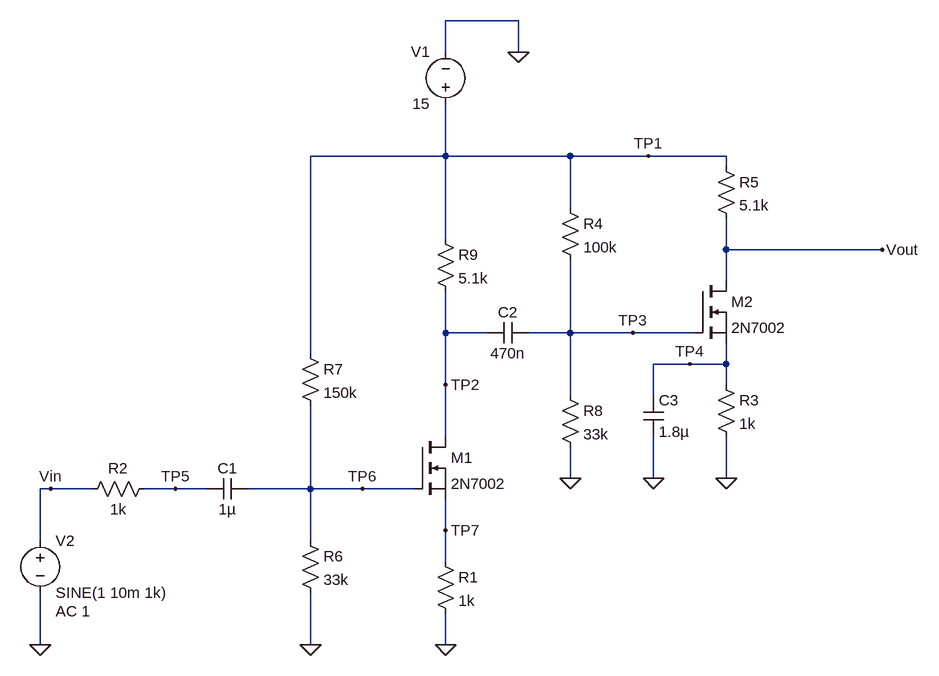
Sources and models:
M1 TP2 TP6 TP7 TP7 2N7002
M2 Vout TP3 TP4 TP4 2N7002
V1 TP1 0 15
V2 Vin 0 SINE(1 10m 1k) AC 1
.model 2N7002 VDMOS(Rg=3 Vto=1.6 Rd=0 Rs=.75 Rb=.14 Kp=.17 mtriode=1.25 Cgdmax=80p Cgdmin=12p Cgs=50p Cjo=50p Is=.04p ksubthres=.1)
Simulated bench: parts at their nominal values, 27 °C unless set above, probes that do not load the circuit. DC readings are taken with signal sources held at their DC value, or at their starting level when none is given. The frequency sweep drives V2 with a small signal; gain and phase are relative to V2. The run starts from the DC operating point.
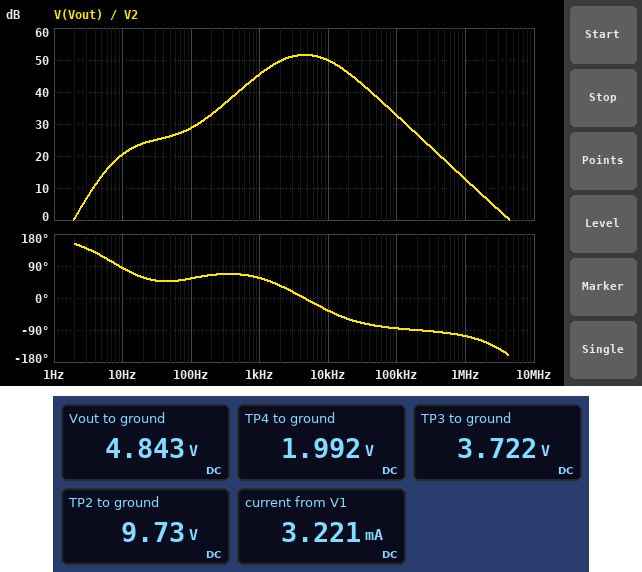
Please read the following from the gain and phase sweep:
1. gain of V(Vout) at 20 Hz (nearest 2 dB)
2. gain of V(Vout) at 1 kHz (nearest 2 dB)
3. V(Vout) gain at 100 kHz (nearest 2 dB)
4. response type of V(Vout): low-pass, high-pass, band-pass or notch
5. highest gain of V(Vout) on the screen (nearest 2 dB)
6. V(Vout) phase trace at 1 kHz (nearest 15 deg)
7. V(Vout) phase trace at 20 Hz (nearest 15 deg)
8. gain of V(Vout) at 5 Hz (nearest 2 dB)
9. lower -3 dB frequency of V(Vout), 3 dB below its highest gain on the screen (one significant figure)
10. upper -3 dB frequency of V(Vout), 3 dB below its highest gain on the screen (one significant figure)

24 dB
46 dB
32 dB
band-pass
52 dB
60 deg
60 deg
14 dB
2 kHz
10 kHz
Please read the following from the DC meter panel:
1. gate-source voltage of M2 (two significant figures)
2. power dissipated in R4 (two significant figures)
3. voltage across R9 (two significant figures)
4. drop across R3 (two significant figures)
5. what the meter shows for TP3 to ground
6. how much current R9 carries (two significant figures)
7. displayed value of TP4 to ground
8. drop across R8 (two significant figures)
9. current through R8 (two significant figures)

1.7 V
1.3 mW
5.3 V
2.0 V
3.722 V
1.0 mA
1.992 V
3.7 V
110 µA
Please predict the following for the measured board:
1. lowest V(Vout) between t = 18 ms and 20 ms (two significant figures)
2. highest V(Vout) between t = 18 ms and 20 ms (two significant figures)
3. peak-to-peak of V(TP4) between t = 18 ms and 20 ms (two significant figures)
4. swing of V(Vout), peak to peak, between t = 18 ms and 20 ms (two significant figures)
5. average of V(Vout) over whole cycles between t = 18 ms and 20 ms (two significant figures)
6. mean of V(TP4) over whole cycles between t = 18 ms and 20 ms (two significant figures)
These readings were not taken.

2.9 V
6.7 V
66 mV
3.8 V
4.8 V
2.0 V
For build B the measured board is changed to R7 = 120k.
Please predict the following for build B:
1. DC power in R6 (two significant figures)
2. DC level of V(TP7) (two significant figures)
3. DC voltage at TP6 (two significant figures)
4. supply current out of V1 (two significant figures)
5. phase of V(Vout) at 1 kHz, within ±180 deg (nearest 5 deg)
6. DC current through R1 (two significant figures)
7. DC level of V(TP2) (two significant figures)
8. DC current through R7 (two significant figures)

320 µW
1.5 V
3.2 V
3.7 mA
55 deg
1.5 mA
7.2 V
98 µA
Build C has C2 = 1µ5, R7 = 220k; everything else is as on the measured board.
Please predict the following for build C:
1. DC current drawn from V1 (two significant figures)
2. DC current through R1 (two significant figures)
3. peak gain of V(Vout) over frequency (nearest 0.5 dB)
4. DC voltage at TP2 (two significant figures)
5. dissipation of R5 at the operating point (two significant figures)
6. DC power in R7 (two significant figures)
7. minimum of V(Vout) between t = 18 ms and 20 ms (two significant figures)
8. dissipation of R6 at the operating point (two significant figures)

2.5 mA
360 µA
51.0 dB
13 V
20 mW
770 µW
3.0 V
120 µW
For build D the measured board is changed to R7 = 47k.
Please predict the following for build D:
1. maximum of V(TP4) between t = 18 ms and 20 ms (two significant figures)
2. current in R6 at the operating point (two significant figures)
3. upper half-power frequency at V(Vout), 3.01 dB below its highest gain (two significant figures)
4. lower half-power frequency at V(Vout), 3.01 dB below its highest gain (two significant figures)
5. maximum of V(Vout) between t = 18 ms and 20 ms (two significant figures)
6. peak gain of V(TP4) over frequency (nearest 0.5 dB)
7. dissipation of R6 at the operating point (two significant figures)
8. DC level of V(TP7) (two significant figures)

2.0 V
190 µA
1.3 MHz
47 kHz
4.8 V
-54.5 dB
1.2 mW
2.5 V
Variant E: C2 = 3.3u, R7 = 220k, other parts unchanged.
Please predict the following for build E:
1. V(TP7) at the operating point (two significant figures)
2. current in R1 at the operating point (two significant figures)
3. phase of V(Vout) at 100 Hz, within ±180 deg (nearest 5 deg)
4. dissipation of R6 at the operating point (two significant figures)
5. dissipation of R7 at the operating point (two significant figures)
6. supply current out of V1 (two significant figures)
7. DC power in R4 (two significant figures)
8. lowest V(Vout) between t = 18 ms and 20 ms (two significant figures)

360 mV
360 µA
50 deg
120 µW
770 µW
2.5 mA
1.3 mW
3.0 V
